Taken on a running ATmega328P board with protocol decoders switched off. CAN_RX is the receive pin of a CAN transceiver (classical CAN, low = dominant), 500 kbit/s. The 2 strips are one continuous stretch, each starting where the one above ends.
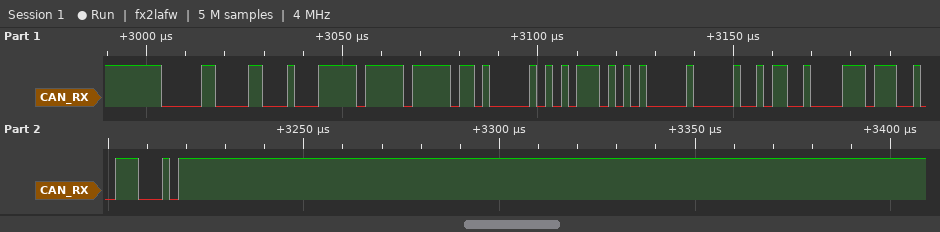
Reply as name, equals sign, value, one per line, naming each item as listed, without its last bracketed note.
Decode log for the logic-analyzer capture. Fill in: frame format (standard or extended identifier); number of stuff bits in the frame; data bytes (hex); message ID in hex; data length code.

frame format = standard
number of stuff bits in the frame = 7
data bytes = FF FF A0 57 54 00 2C 87
message ID in hex = 0x043
data length code = 8
